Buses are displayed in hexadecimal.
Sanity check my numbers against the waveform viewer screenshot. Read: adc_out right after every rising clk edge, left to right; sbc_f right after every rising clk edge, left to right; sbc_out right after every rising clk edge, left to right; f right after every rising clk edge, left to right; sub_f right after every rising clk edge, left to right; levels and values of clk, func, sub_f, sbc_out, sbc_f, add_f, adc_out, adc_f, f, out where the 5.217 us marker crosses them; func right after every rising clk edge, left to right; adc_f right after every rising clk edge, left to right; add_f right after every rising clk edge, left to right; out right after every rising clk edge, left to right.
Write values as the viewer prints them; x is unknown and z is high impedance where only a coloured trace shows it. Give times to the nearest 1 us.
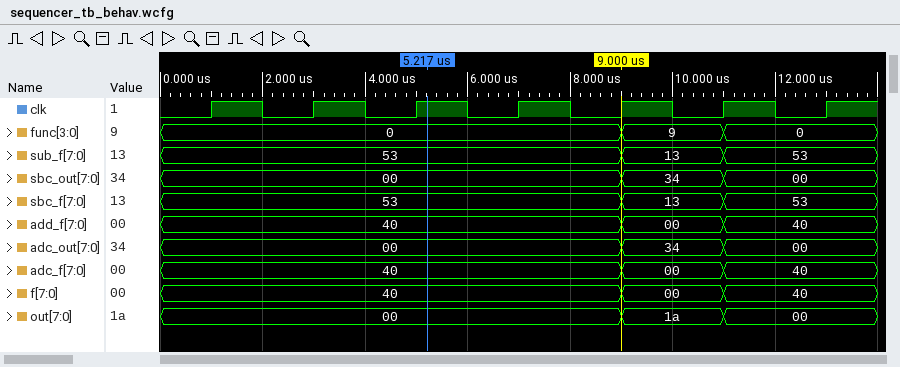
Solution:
00, 00, 00, 00, 34, 00, 00
53, 53, 53, 53, 13, 53, 53
00, 00, 00, 00, 34, 00, 00
40, 40, 40, 40, 00, 40, 40
53, 53, 53, 53, 13, 53, 53
clk=1, func=0, sub_f=53, sbc_out=00, sbc_f=53, add_f=40, adc_out=00, adc_f=40, f=40, out=00
0, 0, 0, 0, 9, 0, 0
40, 40, 40, 40, 00, 40, 40
40, 40, 40, 40, 00, 40, 40
00, 00, 00, 00, 1a, 00, 00
